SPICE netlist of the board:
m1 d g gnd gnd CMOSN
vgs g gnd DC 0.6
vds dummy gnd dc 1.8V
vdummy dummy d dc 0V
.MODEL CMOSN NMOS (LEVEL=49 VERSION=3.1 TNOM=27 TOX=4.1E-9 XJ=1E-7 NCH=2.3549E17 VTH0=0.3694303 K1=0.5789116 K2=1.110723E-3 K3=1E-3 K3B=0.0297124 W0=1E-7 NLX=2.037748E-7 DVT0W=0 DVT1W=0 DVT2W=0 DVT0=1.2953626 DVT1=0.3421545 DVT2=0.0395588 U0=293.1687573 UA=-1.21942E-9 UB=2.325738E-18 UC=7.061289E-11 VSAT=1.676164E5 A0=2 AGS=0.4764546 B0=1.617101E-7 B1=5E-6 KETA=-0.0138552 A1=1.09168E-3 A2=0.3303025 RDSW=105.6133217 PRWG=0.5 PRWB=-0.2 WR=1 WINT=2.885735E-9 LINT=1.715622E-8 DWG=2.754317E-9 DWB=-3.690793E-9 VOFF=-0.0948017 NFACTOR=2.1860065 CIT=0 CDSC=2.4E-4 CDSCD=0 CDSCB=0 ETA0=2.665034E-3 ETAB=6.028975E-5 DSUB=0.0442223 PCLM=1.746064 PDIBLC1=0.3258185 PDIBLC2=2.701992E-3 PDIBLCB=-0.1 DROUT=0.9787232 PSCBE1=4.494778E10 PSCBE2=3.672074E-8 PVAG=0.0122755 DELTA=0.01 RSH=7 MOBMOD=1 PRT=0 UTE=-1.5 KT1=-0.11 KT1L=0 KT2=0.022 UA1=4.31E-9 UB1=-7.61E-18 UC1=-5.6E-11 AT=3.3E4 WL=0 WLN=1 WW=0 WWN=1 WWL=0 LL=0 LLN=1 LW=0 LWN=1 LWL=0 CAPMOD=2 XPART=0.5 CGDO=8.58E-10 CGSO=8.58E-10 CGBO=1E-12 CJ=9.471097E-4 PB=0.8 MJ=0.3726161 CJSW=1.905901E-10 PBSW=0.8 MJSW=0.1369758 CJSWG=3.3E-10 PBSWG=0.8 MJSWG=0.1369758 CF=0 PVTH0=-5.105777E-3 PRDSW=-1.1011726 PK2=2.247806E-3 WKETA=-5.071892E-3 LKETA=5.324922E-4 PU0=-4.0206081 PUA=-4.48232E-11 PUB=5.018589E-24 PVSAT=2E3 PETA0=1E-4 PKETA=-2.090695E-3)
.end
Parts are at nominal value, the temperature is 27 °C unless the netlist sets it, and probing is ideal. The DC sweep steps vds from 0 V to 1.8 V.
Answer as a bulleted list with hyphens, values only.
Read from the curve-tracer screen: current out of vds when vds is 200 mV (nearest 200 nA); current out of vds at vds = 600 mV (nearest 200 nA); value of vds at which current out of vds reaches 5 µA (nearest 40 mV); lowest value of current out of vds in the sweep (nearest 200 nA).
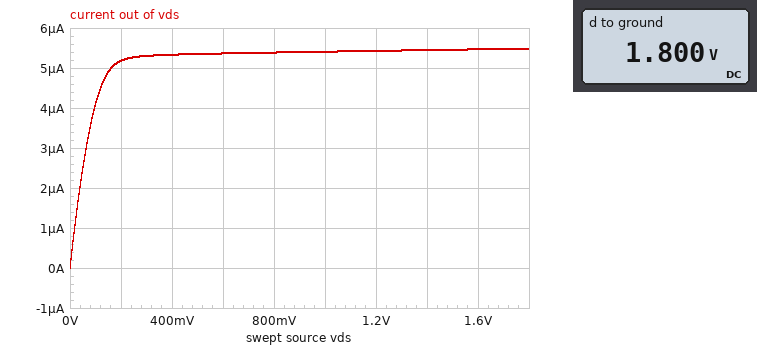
- 5.2 µA
- 5.4 µA
- 160 mV
- 0 A
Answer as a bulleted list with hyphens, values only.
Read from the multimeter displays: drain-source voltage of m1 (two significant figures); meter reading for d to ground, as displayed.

- 1.8 V
- 1.800 V
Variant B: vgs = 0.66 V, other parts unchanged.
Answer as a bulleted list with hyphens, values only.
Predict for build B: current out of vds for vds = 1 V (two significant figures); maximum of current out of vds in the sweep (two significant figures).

- 8.8 µA
- 8.9 µA
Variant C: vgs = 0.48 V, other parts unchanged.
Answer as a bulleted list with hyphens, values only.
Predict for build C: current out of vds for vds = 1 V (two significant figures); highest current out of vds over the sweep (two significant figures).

- 1.2 µA
- 1.3 µA
